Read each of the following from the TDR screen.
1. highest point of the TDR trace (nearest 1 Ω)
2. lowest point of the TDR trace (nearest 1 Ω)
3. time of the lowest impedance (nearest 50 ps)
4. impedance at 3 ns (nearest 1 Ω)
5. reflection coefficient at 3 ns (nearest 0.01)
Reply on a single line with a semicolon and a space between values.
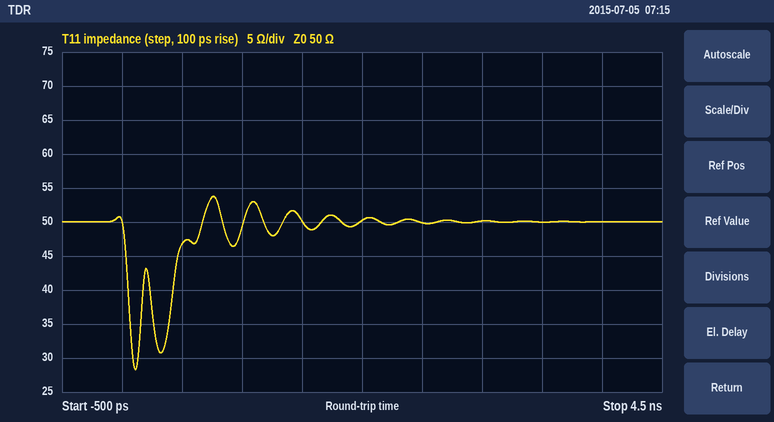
54 Ω; 28 Ω; 100 ps; 50 Ω; 0.00
